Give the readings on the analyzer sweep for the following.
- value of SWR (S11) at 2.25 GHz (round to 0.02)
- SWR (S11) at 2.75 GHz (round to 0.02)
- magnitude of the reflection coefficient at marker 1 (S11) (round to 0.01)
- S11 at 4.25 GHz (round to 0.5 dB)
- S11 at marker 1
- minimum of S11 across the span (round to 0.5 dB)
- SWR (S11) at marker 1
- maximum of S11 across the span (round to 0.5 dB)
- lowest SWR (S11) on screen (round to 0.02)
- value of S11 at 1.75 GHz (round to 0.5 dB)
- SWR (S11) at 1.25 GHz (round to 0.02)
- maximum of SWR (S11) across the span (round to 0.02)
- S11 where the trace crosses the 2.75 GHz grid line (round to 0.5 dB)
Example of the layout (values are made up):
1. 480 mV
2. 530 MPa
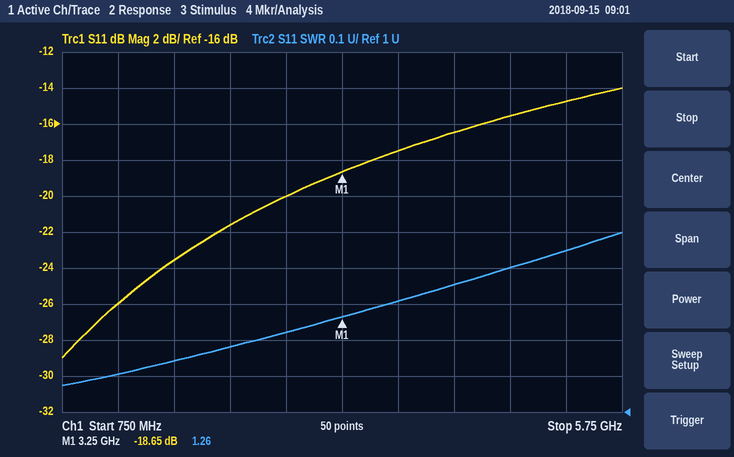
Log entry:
1. 1.18
2. 1.22
3. 0.12
4. -16.5 dB
5. -18.65 dB
6. -29.0 dB
7. 1.26
8. -14.0 dB
9. 1.08
10. -23.5 dB
11. 1.10
12. 1.50
13. -20.0 dB
